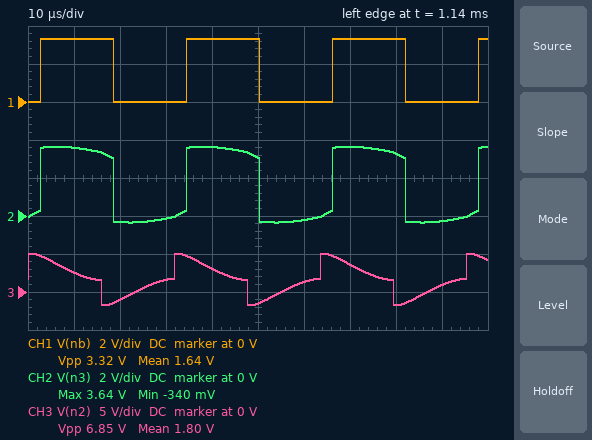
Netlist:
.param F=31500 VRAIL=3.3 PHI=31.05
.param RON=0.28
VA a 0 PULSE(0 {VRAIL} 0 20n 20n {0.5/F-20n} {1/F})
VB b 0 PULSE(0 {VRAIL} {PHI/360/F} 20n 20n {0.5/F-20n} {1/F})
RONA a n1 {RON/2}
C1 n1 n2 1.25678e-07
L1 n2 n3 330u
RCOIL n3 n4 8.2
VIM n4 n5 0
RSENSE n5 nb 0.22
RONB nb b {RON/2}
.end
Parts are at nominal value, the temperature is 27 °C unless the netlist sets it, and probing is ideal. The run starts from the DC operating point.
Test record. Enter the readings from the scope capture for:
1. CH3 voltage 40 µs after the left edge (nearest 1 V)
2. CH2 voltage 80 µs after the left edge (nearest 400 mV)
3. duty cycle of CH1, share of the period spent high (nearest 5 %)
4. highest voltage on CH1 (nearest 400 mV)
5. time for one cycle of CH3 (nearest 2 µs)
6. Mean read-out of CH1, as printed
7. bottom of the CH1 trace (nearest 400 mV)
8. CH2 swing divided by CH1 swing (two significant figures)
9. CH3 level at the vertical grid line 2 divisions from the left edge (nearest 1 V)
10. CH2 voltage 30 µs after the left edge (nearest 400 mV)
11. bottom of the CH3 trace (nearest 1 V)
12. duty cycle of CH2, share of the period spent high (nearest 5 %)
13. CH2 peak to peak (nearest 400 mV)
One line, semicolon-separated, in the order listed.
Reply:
3 V; 3.2 V; 50 %; 3.2 V; 32 µs; 1.64 V; 0 V; 1.2; -1 V; 0 V; -2 V; 50 %; 4.0 V
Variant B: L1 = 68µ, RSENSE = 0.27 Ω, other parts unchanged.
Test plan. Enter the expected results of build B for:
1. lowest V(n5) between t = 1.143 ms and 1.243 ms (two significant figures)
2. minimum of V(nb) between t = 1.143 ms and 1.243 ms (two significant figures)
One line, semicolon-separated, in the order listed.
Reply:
-25 mV; -8.6 mV
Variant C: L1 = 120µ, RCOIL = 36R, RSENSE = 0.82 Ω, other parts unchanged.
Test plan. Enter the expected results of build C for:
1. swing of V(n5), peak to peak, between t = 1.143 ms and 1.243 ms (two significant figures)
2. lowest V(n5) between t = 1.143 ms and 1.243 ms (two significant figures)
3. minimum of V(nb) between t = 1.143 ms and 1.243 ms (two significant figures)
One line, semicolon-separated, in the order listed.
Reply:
3.4 V; -48 mV; -7.0 mV
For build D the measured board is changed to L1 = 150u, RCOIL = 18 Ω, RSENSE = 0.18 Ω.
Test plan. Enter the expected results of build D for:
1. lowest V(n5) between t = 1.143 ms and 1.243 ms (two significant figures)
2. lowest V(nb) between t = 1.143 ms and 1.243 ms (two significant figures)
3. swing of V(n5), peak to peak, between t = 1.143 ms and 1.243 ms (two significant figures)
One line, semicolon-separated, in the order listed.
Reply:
-19 mV; -8.5 mV; 3.3 V
